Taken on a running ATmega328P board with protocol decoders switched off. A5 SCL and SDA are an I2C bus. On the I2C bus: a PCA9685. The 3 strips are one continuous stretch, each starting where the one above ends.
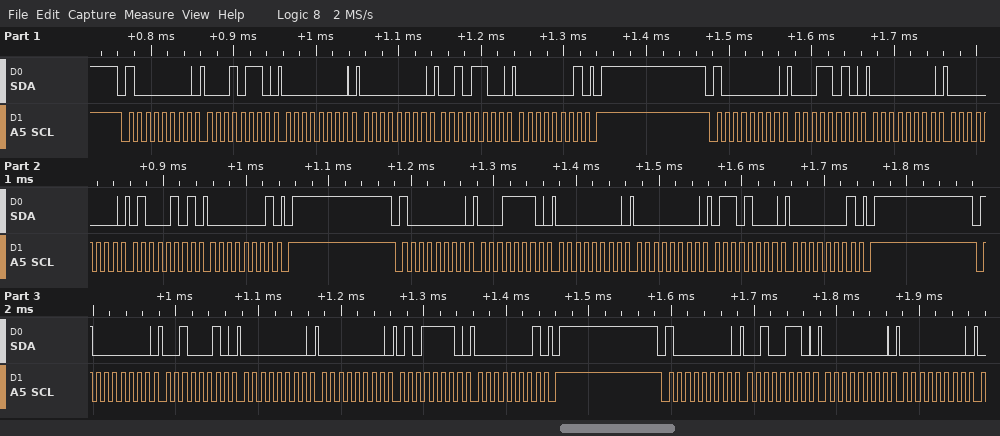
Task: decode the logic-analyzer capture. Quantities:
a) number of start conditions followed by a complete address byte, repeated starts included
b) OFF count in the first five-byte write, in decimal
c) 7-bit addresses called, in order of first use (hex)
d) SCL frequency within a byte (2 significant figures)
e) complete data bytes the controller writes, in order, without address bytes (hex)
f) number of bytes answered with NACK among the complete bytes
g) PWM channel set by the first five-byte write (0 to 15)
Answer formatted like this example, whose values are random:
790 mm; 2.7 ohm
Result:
5; 300; 0x40; 100 kHz; 16 00 00 2C 01 1A 00 00 45 01 1E 00 00 68 01 22 00 00 5E 01 26 00 00; 0; 4
